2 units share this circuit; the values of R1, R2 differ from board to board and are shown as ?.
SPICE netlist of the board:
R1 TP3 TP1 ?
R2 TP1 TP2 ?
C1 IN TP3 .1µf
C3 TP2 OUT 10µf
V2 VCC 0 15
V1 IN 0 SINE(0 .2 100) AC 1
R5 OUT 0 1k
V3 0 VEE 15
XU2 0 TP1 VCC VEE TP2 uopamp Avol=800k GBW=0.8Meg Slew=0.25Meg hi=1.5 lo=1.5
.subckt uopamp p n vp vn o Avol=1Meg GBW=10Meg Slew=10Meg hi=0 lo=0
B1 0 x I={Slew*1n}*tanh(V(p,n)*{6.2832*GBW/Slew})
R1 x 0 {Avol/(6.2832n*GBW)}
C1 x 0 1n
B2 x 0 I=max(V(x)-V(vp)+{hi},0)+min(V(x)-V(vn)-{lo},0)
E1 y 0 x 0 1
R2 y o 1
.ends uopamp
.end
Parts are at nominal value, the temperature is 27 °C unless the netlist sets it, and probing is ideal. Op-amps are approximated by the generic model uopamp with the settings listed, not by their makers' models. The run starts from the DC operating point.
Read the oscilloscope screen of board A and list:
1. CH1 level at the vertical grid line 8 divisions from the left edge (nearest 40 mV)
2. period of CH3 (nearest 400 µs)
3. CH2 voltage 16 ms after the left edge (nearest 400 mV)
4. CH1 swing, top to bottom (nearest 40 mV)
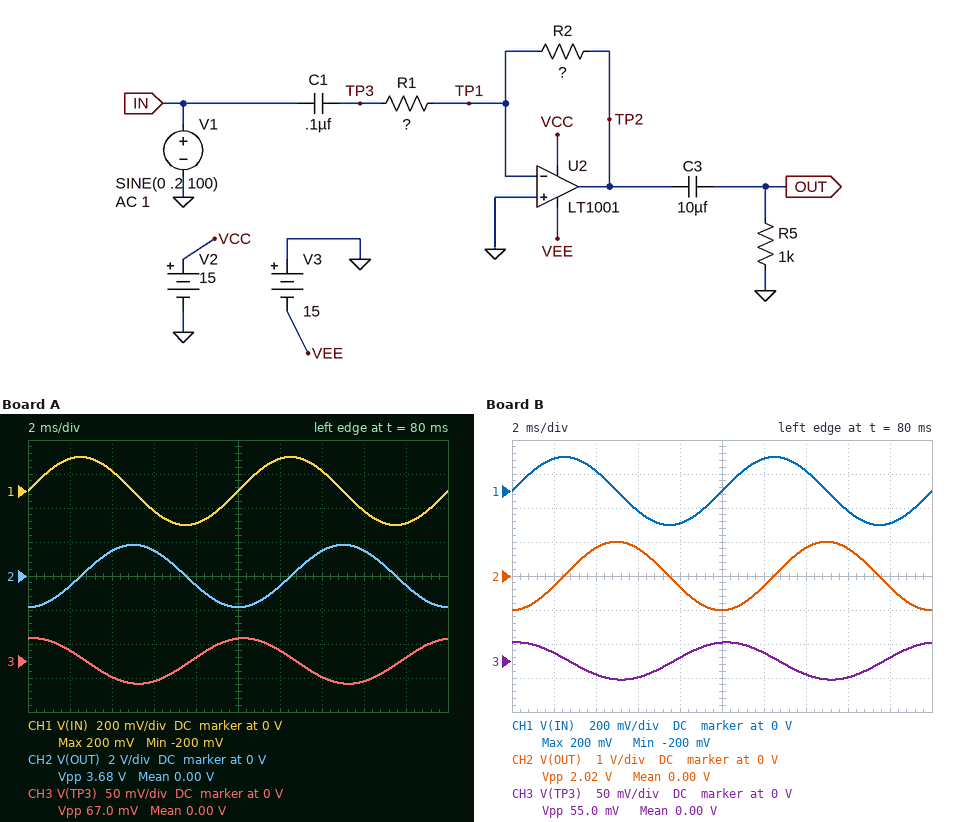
-120 mV
10.0 ms
1.6 V
400 mV
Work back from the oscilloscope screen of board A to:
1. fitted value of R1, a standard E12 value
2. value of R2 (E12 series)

2.7 kΩ
150 kΩ
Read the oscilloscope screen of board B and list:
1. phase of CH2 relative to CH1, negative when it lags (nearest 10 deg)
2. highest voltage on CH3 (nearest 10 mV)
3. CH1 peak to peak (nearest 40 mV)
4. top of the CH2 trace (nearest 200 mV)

-90 deg
30 mV
400 mV
1.0 V
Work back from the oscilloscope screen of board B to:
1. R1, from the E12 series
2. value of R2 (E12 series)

2.2 kΩ
82 kΩ
